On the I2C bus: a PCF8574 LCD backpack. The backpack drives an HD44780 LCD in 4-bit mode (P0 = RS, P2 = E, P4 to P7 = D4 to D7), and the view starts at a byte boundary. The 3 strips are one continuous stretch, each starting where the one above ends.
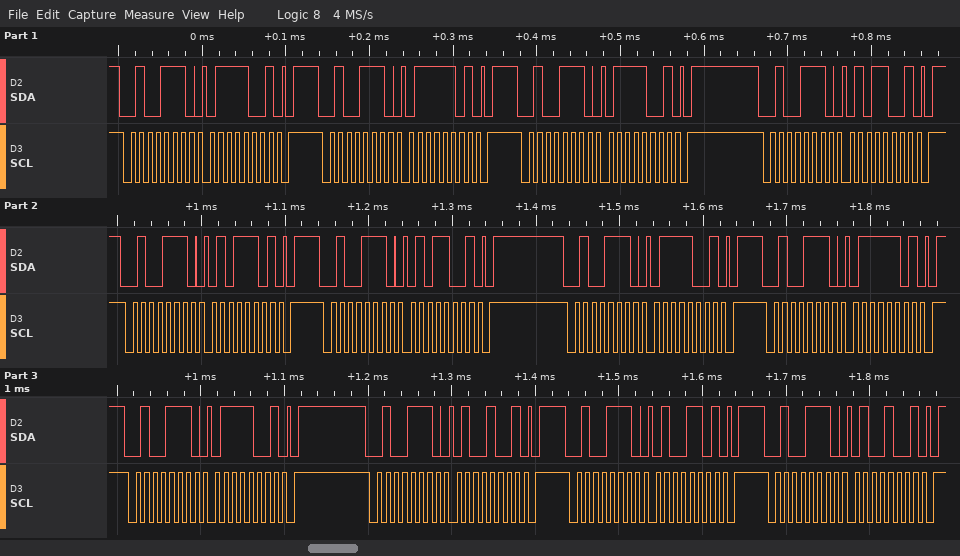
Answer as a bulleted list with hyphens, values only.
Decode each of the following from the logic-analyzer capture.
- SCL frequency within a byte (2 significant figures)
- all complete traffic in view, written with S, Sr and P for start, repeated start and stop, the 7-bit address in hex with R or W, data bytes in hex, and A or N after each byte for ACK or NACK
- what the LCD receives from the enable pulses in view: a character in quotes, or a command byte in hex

- 100 kHz
- S 27W A 79 A P S 27W A 7D A P S 27W A 79 A P S 27W A 59 A P S 27W A 5D A P S 27W A 59 A P S 27W A 79 A P S 27W A 7D A P S 27W A 79 A P S 27W A 49 A P S 27W A 4D A P S 27W A 49 A P
- 'u' 't'
